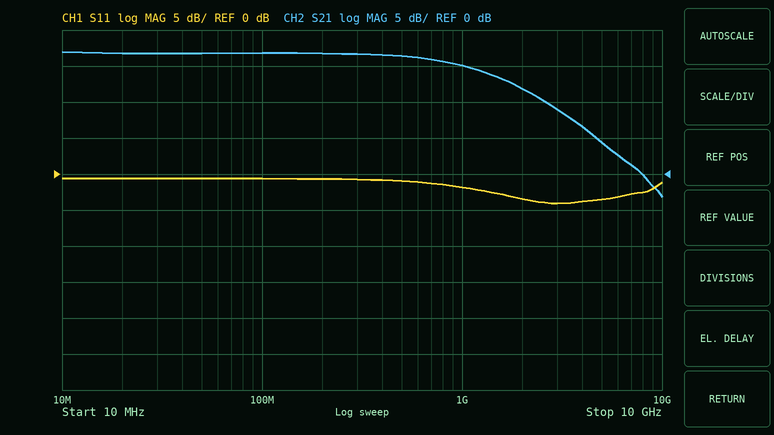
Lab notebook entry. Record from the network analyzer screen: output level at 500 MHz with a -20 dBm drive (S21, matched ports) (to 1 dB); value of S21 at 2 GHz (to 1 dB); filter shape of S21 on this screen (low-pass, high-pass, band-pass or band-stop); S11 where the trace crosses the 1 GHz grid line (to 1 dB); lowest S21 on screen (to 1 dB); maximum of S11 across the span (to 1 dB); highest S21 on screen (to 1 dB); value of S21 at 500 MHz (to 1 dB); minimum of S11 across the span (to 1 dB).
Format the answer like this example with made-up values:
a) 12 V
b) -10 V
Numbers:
a) -4 dBm
b) 12 dB
c) low-pass
d) -2 dB
e) -3 dB
f) -1 dB
g) 17 dB
h) 16 dB
i) -4 dB
